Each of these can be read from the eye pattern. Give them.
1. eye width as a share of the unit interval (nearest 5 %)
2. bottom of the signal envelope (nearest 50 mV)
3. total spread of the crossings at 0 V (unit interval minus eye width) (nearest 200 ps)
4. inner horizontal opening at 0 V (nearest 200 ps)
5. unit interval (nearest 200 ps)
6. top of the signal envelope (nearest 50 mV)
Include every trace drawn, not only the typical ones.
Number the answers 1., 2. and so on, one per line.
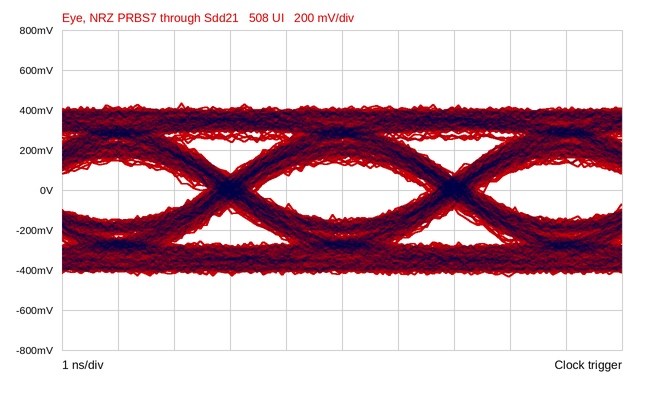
1. 75 %
2. -450 mV
3. 1.0 ns
4. 3.0 ns
5. 4.0 ns
6. 450 mV
